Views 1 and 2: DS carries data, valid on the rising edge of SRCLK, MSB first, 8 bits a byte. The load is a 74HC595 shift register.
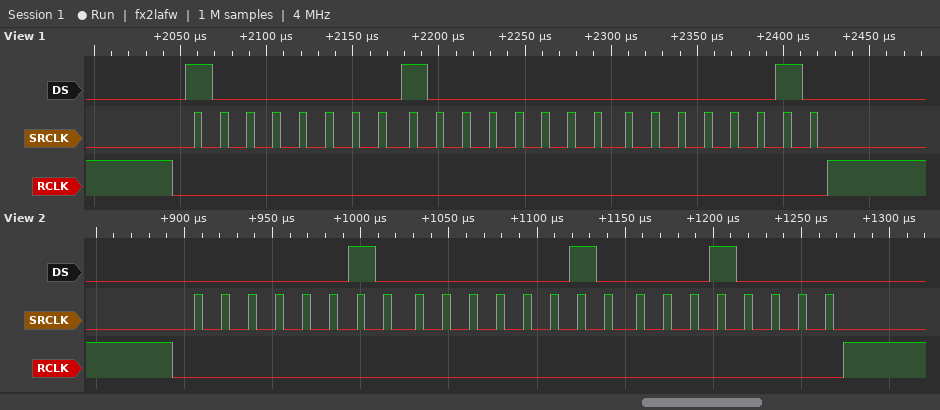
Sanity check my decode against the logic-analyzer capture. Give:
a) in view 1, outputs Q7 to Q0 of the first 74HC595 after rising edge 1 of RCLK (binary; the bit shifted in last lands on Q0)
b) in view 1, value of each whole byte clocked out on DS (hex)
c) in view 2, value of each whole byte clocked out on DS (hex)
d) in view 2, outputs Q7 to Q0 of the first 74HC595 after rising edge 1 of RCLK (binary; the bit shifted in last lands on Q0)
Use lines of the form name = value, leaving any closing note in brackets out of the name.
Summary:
in view 1, outputs Q7 to Q0 of the first 74HC595 after rising edge 1 of RCLK = 00000010
in view 1, value of each whole byte clocked out on DS = 80 80 02
in view 2, value of each whole byte clocked out on DS = 0x02 0x02 0x10
in view 2, outputs Q7 to Q0 of the first 74HC595 after rising edge 1 of RCLK = 00010000
